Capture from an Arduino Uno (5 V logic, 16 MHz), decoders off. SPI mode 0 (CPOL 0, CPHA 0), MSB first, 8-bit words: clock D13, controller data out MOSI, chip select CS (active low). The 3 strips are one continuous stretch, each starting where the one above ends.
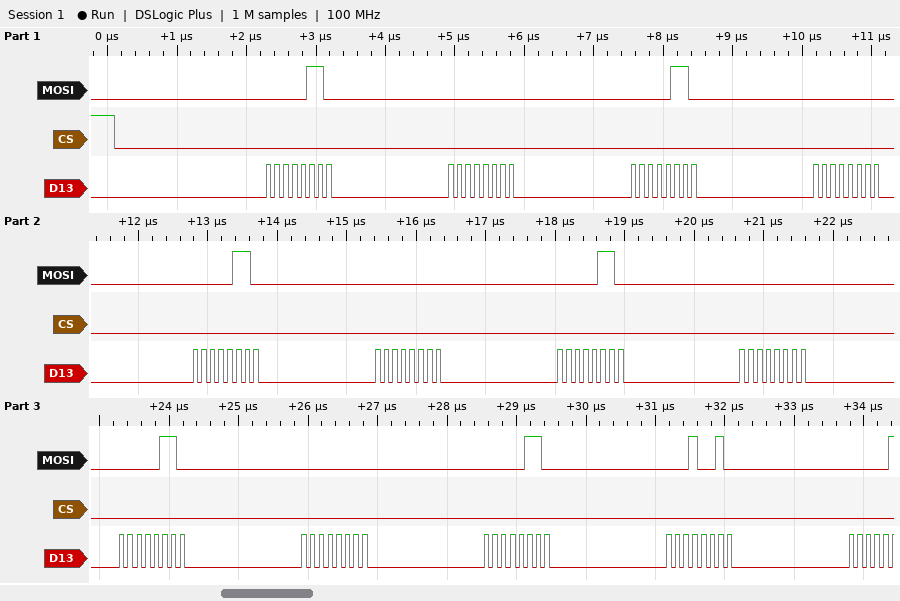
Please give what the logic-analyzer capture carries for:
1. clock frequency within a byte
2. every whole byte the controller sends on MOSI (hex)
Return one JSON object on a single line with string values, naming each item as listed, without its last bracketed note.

{"clock frequency within a byte": "8 MHz", "every whole byte the controller sends on MOSI": "0x06 0x00 0x06 0x00 0x06 0x00 0x06 0x00 0x06 0x00 0x06 0x12"}
